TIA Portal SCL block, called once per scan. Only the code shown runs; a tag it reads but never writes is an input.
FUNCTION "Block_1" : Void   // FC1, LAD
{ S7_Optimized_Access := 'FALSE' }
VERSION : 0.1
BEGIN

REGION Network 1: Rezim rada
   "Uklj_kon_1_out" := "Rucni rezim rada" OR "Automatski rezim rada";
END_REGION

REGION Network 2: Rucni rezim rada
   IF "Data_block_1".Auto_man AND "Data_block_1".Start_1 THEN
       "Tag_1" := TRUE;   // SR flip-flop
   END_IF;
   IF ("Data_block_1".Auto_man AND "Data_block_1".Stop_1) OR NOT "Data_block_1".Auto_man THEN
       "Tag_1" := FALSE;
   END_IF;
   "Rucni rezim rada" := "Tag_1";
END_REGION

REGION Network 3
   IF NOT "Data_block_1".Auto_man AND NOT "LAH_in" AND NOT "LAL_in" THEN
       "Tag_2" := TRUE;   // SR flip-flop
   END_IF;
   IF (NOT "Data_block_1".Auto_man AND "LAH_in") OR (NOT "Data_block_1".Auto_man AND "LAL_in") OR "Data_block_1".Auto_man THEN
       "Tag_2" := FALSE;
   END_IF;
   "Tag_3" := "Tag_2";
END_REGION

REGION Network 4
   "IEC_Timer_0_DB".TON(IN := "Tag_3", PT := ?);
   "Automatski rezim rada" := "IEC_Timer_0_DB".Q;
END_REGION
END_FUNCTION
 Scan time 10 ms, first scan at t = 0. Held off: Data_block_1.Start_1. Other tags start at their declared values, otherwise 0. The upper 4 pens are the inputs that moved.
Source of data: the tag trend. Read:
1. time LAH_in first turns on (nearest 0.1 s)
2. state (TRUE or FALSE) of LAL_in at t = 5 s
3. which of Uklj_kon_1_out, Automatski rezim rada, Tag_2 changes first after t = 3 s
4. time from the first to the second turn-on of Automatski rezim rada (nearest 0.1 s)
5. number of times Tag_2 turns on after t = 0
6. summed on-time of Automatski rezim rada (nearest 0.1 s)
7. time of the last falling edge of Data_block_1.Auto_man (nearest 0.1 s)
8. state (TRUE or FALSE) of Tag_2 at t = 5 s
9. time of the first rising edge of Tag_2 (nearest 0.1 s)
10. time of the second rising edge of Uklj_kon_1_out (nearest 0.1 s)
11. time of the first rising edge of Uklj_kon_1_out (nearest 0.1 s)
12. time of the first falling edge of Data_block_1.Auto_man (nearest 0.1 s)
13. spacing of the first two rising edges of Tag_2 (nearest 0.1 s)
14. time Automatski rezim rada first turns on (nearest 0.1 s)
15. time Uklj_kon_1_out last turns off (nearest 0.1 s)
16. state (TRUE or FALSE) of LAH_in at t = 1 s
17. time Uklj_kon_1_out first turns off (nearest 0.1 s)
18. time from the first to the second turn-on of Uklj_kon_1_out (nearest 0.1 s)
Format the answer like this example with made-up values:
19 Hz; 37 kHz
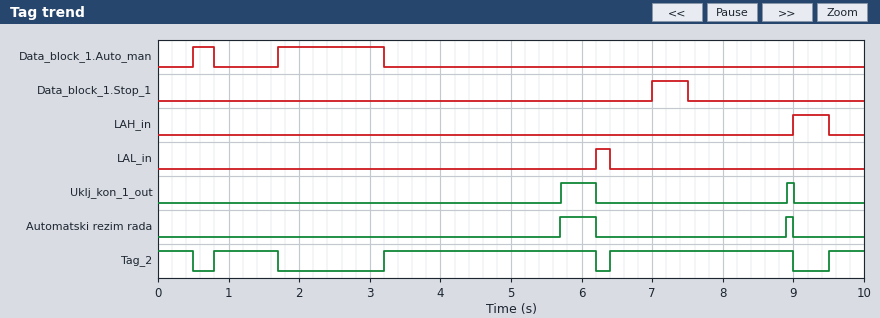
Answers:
9.0 s; FALSE; Tag_2; 3.2 s; 4; 0.6 s; 3.2 s; TRUE; 0.8 s; 8.9 s; 5.7 s; 0.8 s; 2.4 s; 5.7 s; 9.0 s; FALSE; 6.2 s; 3.2 s
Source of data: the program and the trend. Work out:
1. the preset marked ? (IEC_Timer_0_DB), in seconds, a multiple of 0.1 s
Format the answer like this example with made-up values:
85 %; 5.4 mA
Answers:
2.5 s
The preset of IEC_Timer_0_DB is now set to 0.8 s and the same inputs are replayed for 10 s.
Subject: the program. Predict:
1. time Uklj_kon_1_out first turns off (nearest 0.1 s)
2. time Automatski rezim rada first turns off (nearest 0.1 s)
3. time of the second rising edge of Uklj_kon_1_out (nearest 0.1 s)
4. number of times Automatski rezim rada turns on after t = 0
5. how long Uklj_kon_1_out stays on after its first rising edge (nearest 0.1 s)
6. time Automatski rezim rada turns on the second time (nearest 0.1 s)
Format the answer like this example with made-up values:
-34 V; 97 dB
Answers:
1.7 s; 1.7 s; 4.0 s; 3; 0.1 s; 4.0 s
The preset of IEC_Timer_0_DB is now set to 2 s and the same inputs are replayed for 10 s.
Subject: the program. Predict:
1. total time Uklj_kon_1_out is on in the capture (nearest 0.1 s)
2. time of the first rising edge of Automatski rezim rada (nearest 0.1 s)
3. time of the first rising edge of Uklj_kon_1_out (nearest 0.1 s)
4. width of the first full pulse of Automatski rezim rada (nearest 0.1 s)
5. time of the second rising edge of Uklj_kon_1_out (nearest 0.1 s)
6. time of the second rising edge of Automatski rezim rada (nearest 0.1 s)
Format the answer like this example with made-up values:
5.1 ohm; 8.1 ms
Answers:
1.6 s; 5.2 s; 5.2 s; 1.0 s; 8.4 s; 8.4 s
